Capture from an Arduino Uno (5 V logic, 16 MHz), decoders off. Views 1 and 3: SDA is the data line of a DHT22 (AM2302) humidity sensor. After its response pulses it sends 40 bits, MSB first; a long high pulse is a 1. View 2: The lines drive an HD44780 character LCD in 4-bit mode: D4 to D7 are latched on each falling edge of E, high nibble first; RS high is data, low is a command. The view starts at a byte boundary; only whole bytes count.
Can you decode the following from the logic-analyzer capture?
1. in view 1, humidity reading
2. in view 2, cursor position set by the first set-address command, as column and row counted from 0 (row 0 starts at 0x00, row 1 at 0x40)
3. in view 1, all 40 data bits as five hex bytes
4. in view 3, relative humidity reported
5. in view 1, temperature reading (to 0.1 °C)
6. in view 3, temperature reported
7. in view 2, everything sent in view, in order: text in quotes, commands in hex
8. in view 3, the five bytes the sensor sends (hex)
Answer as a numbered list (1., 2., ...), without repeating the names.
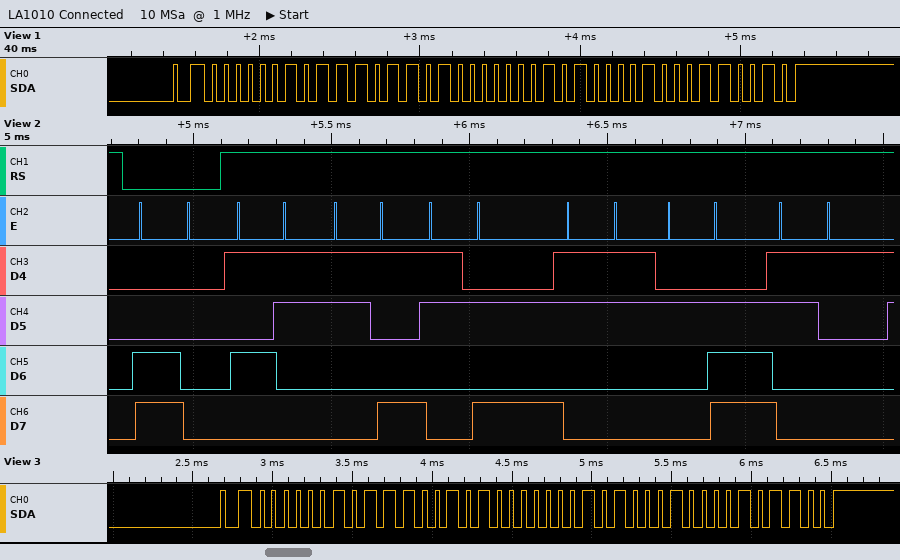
1. 74.9 %
2. column 0, row 1
3. 02 ED 01 42 32
4. 74.1 %
5. 32.2 °C
6. 32.4 °C
7. 0xC0 "S9:3.1"
8. 02 E5 01 44 2C
